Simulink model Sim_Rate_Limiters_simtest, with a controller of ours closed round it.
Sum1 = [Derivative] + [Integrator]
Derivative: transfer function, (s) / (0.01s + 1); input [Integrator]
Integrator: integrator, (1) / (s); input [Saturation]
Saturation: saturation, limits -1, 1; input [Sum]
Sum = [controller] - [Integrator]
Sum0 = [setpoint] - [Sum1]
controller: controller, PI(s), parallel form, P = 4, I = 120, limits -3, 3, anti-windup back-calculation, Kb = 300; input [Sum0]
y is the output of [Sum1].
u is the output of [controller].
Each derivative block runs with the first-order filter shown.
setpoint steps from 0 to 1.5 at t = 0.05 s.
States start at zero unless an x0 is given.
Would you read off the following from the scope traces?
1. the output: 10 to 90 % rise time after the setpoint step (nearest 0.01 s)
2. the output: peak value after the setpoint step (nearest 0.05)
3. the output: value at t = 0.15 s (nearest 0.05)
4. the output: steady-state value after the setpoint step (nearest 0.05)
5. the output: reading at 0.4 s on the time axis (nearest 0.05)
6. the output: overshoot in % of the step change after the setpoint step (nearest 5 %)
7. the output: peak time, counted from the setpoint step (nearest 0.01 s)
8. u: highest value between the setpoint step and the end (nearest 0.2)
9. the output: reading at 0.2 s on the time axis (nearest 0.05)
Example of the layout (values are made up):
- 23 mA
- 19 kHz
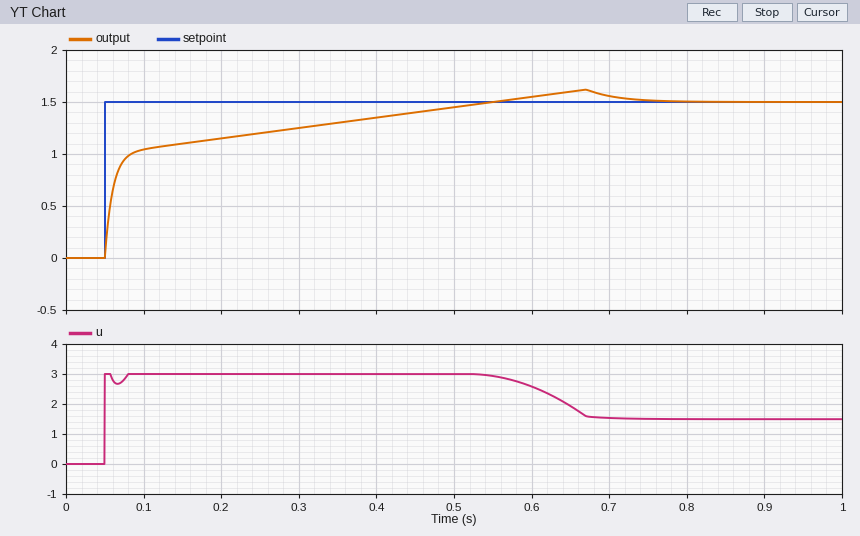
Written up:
- 0.35 s
- 1.60
- 1.10
- 1.50
- 1.35
- 10 %
- 0.62 s
- 3.0
- 1.15
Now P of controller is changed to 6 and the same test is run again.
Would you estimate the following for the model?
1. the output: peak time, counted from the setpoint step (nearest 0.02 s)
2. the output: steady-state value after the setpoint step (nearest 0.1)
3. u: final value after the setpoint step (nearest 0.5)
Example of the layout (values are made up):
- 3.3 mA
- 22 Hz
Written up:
- 0.60 s
- 1.5
- 1.5
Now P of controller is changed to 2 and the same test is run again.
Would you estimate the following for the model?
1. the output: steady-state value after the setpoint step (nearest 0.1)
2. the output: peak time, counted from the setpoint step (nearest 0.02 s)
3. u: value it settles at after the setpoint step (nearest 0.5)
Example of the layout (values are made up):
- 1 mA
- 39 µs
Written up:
- 1.5
- 0.64 s
- 1.5
